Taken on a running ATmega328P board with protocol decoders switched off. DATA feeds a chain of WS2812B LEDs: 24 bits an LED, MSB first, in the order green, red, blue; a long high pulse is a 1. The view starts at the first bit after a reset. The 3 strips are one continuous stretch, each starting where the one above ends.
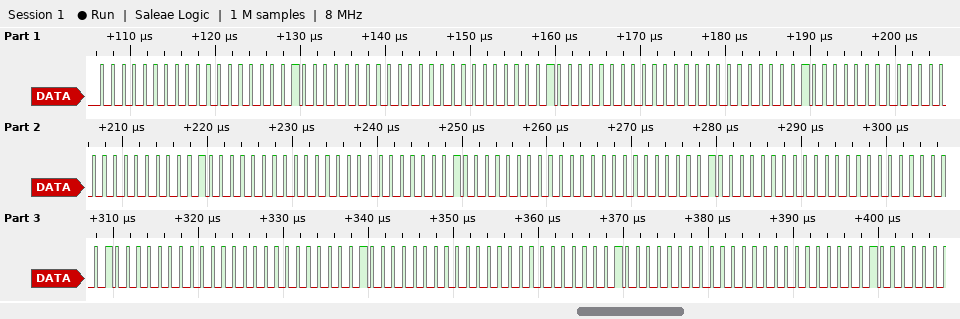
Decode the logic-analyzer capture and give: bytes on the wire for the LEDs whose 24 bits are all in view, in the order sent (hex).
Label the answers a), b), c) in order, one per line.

a) 00 00 20 00 00 20 00 00 20 00 00 20 00 00 20 00 00 20 00 00 20 00 00 20 00 00 20 00 00 20
